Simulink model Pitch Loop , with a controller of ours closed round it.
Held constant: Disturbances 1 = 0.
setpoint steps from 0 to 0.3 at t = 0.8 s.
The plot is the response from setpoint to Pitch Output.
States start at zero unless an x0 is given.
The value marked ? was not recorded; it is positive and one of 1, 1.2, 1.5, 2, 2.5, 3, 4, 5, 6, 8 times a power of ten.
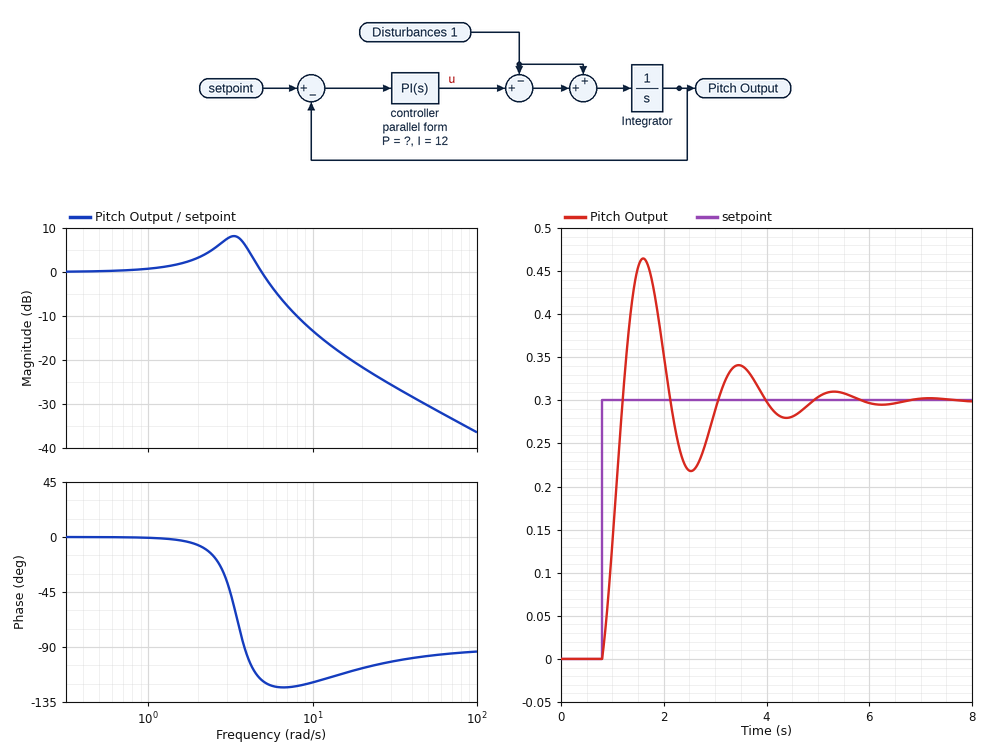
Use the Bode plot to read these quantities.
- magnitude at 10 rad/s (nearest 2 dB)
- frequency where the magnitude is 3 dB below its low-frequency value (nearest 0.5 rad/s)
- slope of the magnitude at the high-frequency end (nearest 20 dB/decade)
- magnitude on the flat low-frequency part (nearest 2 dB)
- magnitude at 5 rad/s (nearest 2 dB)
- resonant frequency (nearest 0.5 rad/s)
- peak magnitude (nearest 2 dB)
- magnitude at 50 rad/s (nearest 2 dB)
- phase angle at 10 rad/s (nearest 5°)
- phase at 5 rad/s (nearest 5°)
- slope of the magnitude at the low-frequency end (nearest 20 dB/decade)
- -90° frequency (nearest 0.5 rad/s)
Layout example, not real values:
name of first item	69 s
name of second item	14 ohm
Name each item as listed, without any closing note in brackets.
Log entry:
magnitude at 10 rad/s	-14 dB
frequency where the magnitude is 3 dB below its low-frequency value	5.5 rad/s
slope of the magnitude at the high-frequency end	-20 dB/decade
magnitude on the flat low-frequency part	0 dB
magnitude at 5 rad/s	0 dB
resonant frequency	3.5 rad/s
peak magnitude	8 dB
magnitude at 50 rad/s	-30 dB
phase angle at 10 rad/s	-120°
phase at 5 rad/s	-120°
slope of the magnitude at the low-frequency end	0 dB/decade
-90° frequency	4.0 rad/s
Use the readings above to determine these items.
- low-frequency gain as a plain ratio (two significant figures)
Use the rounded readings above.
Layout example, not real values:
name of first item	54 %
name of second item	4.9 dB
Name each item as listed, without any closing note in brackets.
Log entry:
low-frequency gain as a plain ratio	1.0
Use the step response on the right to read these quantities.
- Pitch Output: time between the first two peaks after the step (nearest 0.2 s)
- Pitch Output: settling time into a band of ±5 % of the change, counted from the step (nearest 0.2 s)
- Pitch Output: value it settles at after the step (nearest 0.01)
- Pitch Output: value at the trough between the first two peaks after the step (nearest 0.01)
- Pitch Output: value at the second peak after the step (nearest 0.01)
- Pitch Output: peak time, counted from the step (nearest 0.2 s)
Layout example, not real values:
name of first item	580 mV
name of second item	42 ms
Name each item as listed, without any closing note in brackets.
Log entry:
Pitch Output: time between the first two peaks after the step	1.8 s
Pitch Output: settling time into a band of ±5 % of the change, counted from the step	3.8 s
Pitch Output: value it settles at after the step	0.30
Pitch Output: value at the trough between the first two peaks after the step	0.22
Pitch Output: value at the second peak after the step	0.34
Pitch Output: peak time, counted from the step	0.8 s
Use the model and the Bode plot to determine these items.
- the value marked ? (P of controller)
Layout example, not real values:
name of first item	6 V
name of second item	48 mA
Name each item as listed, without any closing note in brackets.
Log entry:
the value marked ?	1.5
